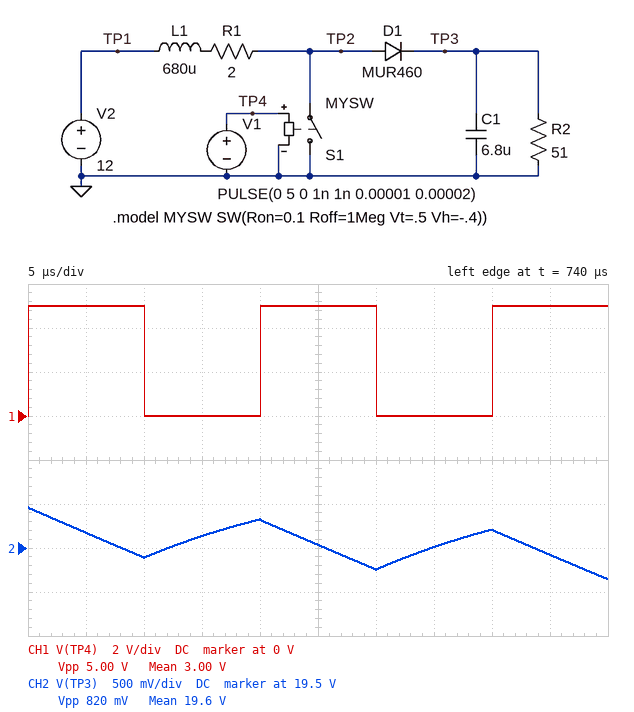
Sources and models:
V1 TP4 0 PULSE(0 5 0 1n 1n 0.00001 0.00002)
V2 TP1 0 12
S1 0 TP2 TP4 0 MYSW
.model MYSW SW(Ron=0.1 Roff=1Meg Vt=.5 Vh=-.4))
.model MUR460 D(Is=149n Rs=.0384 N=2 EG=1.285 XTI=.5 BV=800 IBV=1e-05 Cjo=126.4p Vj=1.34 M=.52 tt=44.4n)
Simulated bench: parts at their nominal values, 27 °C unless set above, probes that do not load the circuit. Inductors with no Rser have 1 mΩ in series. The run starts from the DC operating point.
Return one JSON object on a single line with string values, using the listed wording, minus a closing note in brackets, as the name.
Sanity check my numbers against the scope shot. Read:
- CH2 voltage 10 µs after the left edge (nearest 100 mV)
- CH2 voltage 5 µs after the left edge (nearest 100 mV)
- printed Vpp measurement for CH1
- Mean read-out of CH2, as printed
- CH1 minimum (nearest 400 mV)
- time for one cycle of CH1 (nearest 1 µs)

{"CH2 voltage 10 µs after the left edge": "19.4 V", "CH2 voltage 5 µs after the left edge": "19.7 V", "printed Vpp measurement for CH1": "5.00 V", "Mean read-out of CH2, as printed": "19.6 V", "CH1 minimum": "0 V", "time for one cycle of CH1": "20 µs"}
